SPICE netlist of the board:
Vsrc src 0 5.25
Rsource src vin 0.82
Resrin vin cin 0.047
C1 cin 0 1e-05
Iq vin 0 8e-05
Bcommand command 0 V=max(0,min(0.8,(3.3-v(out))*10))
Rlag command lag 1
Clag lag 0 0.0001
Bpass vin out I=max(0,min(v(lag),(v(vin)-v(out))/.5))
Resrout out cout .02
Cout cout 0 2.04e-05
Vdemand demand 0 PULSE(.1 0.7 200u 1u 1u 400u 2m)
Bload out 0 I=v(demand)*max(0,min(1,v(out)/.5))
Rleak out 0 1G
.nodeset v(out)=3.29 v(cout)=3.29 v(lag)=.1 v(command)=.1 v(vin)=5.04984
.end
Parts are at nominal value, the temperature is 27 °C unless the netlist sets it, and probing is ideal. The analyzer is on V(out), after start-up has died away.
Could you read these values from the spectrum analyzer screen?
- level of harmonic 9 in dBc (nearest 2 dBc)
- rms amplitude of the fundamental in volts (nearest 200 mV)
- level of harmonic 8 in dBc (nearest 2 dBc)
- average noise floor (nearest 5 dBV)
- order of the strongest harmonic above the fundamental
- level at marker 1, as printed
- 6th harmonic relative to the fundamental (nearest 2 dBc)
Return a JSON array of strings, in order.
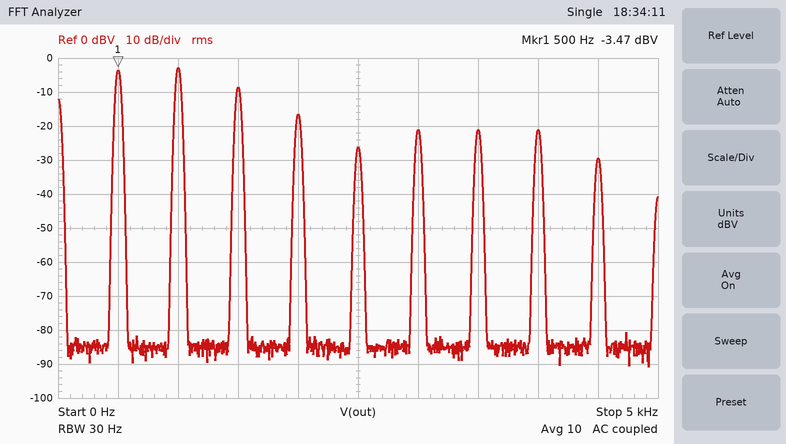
["-26 dBc", "600 mV", "-18 dBc", "-85 dBV", "2", "-3.47 dBV", "-18 dBc"]
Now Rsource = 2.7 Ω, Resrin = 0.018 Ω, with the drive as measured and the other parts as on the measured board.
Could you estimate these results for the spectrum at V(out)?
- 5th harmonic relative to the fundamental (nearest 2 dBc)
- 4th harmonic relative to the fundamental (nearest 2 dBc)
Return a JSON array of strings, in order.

["-30 dBc", "-14 dBc"]
